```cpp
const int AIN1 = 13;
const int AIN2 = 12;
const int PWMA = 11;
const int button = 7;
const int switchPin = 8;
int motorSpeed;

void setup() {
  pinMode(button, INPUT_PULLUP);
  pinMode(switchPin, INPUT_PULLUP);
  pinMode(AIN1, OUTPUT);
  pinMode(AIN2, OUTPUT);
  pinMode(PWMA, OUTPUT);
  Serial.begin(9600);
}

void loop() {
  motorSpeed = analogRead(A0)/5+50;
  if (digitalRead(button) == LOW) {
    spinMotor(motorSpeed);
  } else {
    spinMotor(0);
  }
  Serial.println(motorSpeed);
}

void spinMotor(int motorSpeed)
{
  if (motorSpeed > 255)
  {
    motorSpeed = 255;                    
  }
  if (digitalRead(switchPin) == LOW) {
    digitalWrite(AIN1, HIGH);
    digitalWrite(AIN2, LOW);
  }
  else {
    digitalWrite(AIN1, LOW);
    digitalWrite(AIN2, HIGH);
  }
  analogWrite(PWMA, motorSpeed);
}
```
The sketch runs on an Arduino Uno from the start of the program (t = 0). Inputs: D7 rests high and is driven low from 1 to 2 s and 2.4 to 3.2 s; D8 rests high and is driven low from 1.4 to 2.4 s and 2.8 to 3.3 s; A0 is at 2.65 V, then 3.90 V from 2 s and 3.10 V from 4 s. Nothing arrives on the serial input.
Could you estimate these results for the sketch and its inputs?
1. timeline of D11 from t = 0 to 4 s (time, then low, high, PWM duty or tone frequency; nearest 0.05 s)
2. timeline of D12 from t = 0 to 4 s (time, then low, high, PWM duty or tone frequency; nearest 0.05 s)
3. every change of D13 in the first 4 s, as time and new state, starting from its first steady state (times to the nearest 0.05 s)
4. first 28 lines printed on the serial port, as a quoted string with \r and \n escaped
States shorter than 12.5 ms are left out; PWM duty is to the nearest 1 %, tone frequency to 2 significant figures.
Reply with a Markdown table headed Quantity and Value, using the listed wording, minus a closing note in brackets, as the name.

| Quantity | Value |
|---|---|
| timeline of D11 from t = 0 to 4 s | 0 s low; 1 s PWM 62 %; 2 s low; 2.4 s PWM 82 %; 3.2 s low |
| timeline of D12 from t = 0 to 4 s | 0 s high; 1.4 s low; 2.4 s high; 2.8 s low; 3.3 s high |
| every change of D13 in the first 4 s, as time and new state, starting from its first steady state | 0 s low; 1.4 s high; 2.4 s low; 2.8 s high; 3.3 s low |
| first 28 lines printed on the serial port, as a quoted string with \r and \n escaped | "158\r\n158\r\n158\r\n158\r\n158\r\n158\r\n158\r\n158\r\n158\r\n158\r\n158\r\n158\r\n158\r\n158\r\n158\r\n158\r\n158\r\n158\r\n158\r\n158\r\n158\r\n158\r\n158\r\n158\r\n158\r\n158\r\n158\r\n158\r\n" |
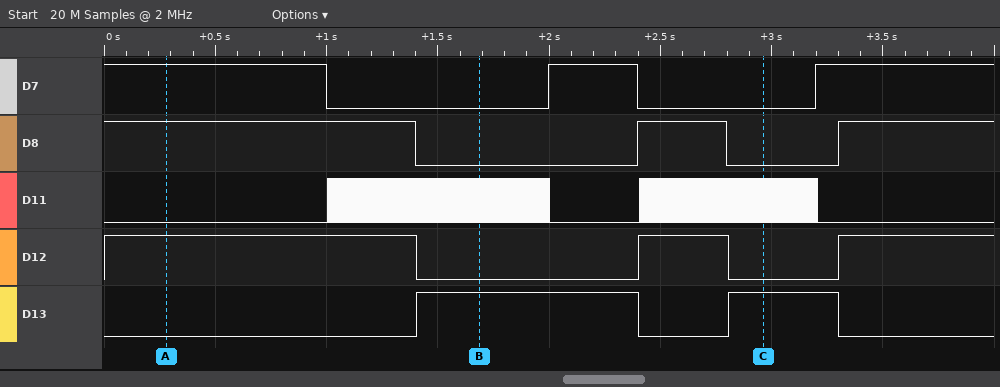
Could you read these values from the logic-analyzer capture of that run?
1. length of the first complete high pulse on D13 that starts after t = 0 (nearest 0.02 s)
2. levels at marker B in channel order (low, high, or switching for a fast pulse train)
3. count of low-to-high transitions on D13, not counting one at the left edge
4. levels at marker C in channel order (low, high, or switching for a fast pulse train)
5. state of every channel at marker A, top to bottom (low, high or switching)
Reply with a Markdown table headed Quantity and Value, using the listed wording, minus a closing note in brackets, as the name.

| Quantity | Value |
|---|---|
| length of the first complete high pulse on D13 that starts after t = 0 | 1.00 s |
| levels at marker B in channel order | D7 low, D8 low, D11 switching, D12 low, D13 high |
| count of low-to-high transitions on D13, not counting one at the left edge | 2 |
| levels at marker C in channel order | D7 low, D8 low, D11 switching, D12 low, D13 high |
| state of every channel at marker A, top to bottom | D7 high, D8 high, D11 low, D12 high, D13 low |
